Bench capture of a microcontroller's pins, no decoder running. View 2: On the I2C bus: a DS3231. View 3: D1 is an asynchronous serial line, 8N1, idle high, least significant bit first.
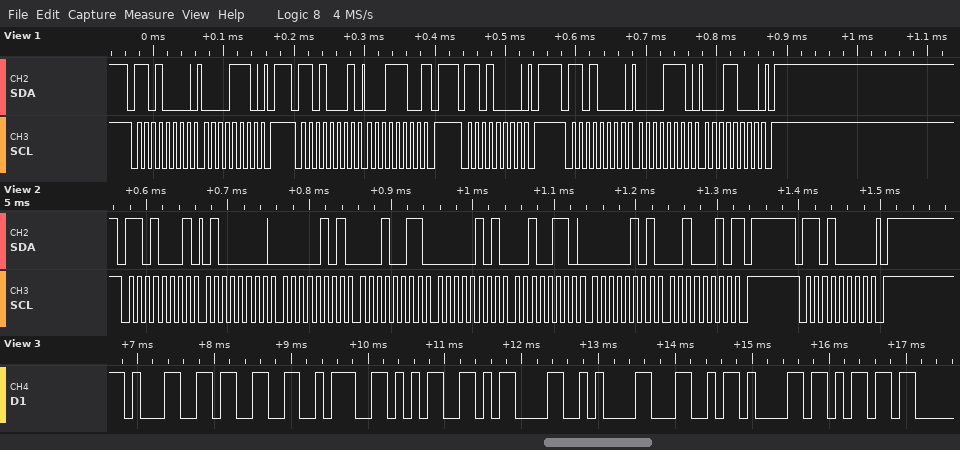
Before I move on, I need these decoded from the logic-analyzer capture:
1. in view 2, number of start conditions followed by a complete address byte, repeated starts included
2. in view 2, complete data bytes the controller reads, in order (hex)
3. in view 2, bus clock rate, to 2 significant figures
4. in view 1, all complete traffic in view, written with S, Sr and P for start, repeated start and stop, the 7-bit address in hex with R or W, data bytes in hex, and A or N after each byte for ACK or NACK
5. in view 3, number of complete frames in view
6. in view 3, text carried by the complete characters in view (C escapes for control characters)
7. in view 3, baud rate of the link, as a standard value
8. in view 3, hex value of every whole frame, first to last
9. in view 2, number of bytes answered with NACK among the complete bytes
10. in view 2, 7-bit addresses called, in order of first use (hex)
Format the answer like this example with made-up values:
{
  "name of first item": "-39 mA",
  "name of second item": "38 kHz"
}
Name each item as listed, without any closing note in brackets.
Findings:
{
  "in view 2, number of start conditions followed by a complete address byte, repeated starts included": "2",
  "in view 2, complete data bytes the controller reads, in order": "40 05 13 05 26 05 22",
  "in view 2, bus clock rate, to 2 significant figures": "100 kHz",
  "in view 1, all complete traffic in view, written with S, Sr and P for start, repeated start and stop, the 7-bit address in hex with R or W, data bytes in hex, and A or N after each byte for ACK or NACK": "S 68W A 0E A P S 68R A 1C N P S 68W A P S 68W A 0E A 18 A P",
  "in view 3, number of complete frames in view": "9",
  "in view 3, text carried by the complete characters in view": "\"13:5\\r\\nLam\"",
  "in view 3, baud rate of the link, as a standard value": "9600 baud",
  "in view 3, hex value of every whole frame, first to last": "31 33 3A 35 0D 0A 4C 61 6D",
  "in view 2, number of bytes answered with NACK among the complete bytes": "1",
  "in view 2, 7-bit addresses called, in order of first use": "0x68"
}
